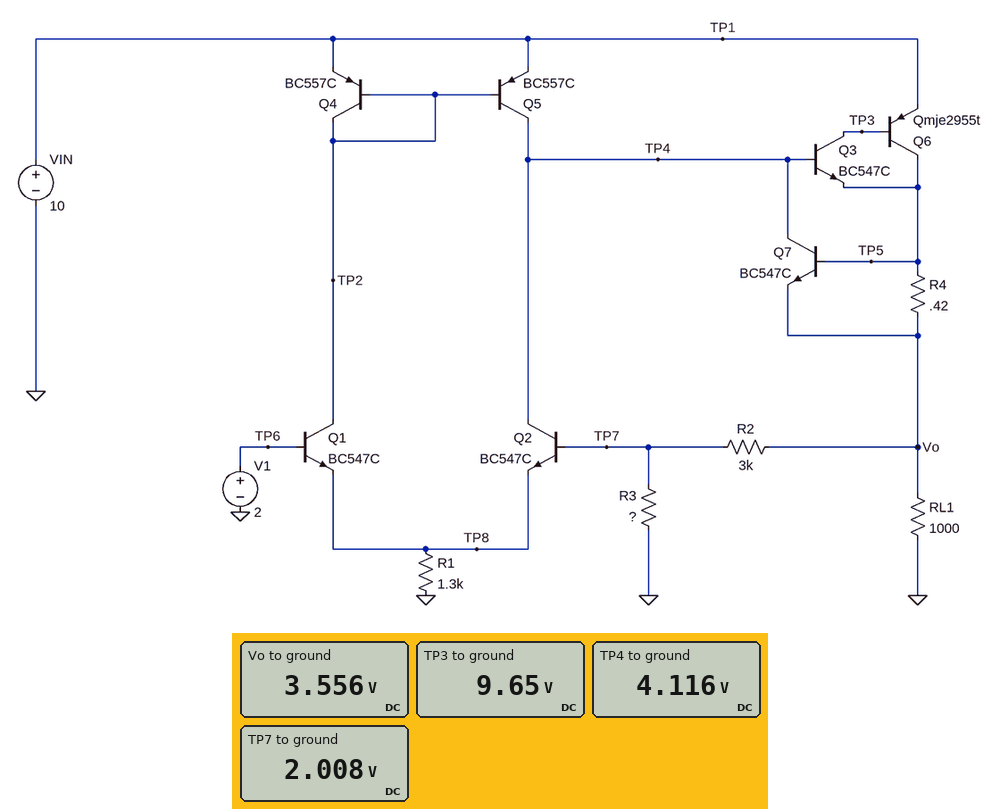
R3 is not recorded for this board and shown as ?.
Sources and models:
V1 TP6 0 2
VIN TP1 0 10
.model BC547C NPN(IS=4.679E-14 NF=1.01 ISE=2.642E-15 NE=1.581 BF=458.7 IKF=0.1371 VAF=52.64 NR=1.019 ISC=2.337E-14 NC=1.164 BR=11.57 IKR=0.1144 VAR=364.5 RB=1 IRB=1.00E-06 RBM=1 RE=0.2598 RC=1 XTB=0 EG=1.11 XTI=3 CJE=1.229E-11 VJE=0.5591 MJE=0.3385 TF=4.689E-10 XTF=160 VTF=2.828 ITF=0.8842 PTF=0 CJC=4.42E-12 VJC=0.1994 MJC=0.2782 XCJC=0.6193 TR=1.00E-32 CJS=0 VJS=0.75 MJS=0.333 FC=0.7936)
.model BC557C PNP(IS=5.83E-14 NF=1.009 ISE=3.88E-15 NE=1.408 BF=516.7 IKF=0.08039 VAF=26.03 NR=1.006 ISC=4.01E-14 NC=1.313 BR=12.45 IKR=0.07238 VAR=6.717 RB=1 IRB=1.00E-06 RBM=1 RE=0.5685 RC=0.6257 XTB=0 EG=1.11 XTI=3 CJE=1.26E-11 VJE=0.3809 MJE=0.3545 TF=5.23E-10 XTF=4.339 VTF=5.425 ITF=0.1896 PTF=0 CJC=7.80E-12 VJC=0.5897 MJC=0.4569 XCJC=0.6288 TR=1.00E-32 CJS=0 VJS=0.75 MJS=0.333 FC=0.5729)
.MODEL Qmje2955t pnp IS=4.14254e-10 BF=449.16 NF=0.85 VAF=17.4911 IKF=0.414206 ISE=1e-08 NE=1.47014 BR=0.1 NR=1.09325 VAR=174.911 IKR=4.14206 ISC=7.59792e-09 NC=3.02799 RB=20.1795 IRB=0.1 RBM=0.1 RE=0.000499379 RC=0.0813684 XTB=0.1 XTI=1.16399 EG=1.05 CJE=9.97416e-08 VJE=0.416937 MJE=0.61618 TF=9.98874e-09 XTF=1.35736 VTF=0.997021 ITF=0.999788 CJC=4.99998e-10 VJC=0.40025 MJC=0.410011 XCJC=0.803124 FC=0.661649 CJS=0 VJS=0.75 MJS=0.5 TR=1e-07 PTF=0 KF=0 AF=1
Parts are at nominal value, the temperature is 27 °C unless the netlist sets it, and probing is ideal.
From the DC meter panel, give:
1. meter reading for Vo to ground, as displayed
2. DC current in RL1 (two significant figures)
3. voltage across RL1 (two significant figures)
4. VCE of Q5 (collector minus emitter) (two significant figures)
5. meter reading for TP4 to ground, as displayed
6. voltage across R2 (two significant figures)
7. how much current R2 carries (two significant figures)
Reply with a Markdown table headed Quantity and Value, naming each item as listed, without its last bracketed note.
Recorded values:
| Quantity | Value |
|---|---|
| meter reading for Vo to ground, as displayed | 3.556 V |
| DC current in RL1 | 3.6 mA |
| voltage across RL1 | 3.6 V |
| VCE of Q5 (collector minus emitter) | -5.9 V |
| meter reading for TP4 to ground, as displayed | 4.116 V |
| voltage across R2 | 1.5 V |
| how much current R2 carries | 520 µA |
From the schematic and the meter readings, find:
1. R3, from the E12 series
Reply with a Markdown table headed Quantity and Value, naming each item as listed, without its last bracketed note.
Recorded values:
| Quantity | Value |
|---|---|
| R3, from the E12 series | 3.9 kΩ |
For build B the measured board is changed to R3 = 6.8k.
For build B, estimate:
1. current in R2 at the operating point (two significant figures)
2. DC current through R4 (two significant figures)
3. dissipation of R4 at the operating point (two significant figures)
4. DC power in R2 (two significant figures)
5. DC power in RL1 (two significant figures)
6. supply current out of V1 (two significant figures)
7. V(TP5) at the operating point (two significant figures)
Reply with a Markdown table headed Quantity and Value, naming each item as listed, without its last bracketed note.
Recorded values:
| Quantity | Value |
|---|---|
| current in R2 at the operating point | 300 µA |
| DC current through R4 | 3.2 mA |
| dissipation of R4 at the operating point | 4.3 µW |
| DC power in R2 | 260 µW |
| DC power in RL1 | 8.4 mW |
| supply current out of V1 | 930 nA |
| V(TP5) at the operating point | 2.9 V |
